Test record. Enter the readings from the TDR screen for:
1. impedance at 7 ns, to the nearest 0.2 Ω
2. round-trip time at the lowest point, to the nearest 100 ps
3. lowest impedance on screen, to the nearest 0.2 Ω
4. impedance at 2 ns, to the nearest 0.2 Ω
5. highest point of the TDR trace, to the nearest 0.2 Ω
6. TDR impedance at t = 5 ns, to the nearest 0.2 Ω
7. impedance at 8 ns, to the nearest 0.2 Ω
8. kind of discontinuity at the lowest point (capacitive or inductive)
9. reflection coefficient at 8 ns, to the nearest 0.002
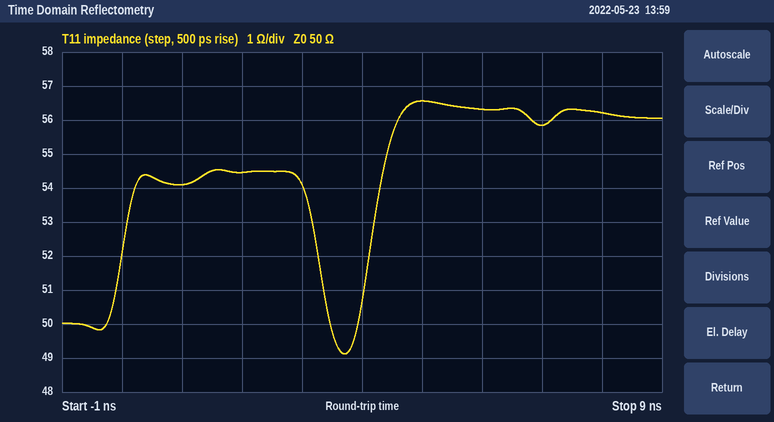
55.8 Ω
3.7 ns
49.2 Ω
54.4 Ω
56.6 Ω
56.6 Ω
56.2 Ω
capacitive
+0.058
